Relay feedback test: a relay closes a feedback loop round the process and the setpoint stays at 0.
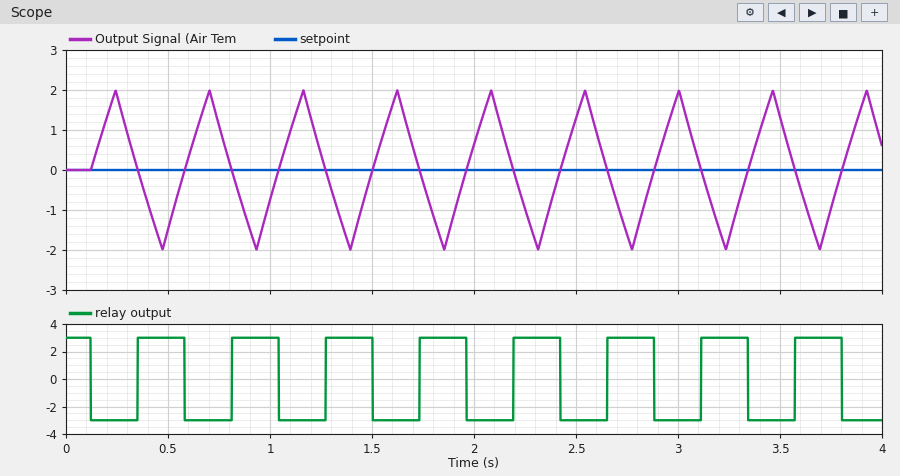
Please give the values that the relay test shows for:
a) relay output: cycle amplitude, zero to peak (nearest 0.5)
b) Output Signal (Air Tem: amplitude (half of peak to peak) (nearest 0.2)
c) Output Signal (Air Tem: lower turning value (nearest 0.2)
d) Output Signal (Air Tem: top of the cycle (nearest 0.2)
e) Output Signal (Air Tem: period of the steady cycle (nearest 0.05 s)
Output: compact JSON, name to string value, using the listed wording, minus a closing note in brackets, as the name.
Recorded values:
{"relay output: cycle amplitude, zero to peak": "3.0", "Output Signal (Air Tem: amplitude (half of peak to peak)": "2.0", "Output Signal (Air Tem: lower turning value": "-2.0", "Output Signal (Air Tem: top of the cycle": "2.0", "Output Signal (Air Tem: period of the steady cycle": "0.45 s"}
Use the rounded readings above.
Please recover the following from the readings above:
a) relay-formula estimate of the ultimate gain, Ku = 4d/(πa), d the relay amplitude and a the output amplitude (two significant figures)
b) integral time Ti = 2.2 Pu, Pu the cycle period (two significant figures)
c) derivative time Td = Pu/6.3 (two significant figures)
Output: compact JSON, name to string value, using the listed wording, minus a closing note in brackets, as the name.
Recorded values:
{"relay-formula estimate of the ultimate gain, Ku = 4d/(πa), d the relay amplitude and a the output amplitude": "1.9", "integral time Ti = 2.2 Pu, Pu the cycle period": "0.99 s", "derivative time Td = Pu/6.3": "0.071 s"}
